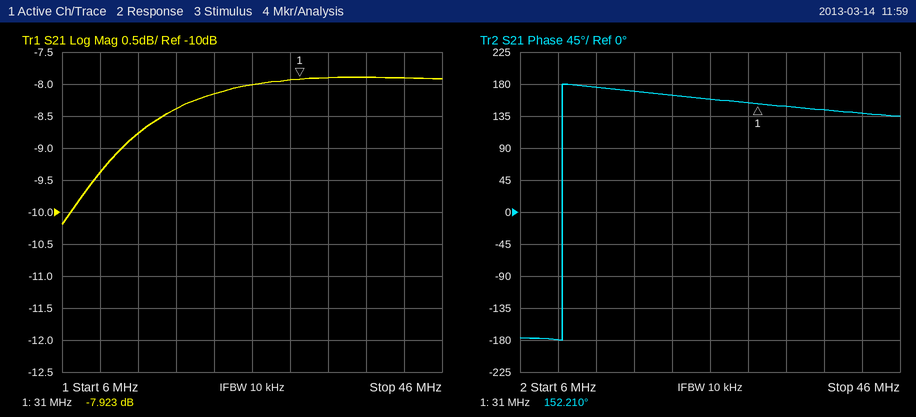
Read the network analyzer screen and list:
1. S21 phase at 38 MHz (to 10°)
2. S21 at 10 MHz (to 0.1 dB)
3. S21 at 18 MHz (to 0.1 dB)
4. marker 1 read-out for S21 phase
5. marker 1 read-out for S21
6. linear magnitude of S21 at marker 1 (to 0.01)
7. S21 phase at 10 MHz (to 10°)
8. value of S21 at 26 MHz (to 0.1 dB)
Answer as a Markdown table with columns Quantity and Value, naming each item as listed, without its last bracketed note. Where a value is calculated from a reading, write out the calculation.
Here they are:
| Quantity | Value |
|---|---|
| S21 phase at 38 MHz | 140° |
| S21 at 10 MHz | -9.4 dB |
| S21 at 18 MHz | -8.4 dB |
| marker 1 read-out for S21 phase | 152.210° |
| marker 1 read-out for S21 | -7.923 dB |
| linear magnitude of S21 at marker 1 | 10^(-7.923/20) ≈ 0.40 |
| S21 phase at 10 MHz | -180° |
| value of S21 at 26 MHz | -8.0 dB |
